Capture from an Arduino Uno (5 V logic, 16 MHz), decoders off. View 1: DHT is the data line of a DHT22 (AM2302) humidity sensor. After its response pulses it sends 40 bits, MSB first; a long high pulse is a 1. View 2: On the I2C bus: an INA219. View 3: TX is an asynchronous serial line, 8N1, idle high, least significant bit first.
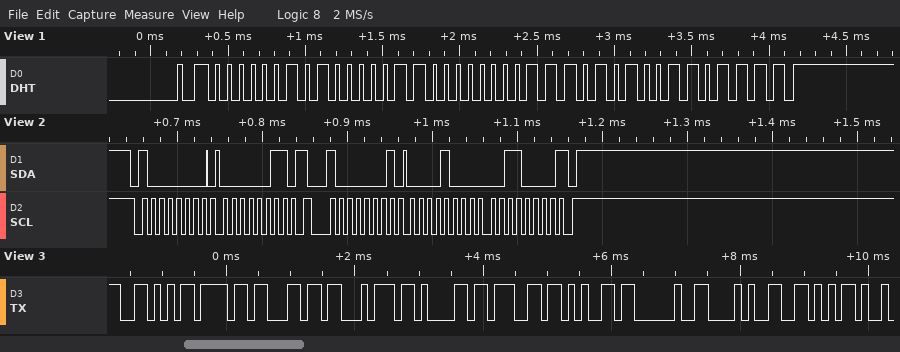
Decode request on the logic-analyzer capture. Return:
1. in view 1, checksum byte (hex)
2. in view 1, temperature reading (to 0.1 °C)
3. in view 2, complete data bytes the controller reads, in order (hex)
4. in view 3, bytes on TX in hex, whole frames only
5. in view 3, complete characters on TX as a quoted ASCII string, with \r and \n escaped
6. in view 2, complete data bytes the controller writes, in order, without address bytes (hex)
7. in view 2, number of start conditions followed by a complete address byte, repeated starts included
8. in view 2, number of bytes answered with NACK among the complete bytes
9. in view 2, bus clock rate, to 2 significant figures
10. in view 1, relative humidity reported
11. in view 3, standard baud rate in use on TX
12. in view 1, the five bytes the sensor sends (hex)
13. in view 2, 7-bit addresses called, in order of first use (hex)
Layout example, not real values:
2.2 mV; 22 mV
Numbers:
0x6F; 23.4 °C; 08 30; 56 6F 6C 74 61 67 65 20 28 56; "Voltage (V"; 03; 2; 1; 100 kHz; 64.3 %; 9600 baud; 02 83 00 EA 6F; 0x40
